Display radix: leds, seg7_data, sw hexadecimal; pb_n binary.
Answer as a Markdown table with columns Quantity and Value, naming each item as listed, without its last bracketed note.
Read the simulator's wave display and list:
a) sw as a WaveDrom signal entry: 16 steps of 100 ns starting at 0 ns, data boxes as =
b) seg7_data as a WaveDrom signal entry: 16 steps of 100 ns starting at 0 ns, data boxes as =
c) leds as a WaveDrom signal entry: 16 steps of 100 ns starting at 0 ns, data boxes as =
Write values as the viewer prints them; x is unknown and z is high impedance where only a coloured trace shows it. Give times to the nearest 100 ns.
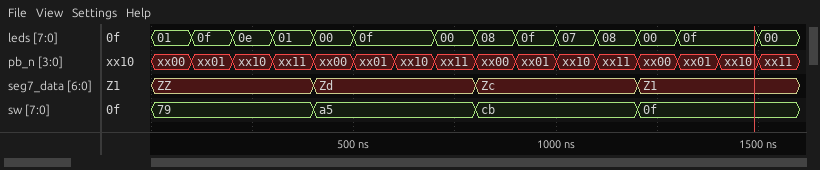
| Quantity | Value |
|---|---|
| sw as a WaveDrom signal entry: 16 steps of 100 ns starting at 0 ns, data boxes as = | {name: 'sw', wave: '=...=...=...=...', data: '79 a5 cb 0f'} |
| seg7_data as a WaveDrom signal entry: 16 steps of 100 ns starting at 0 ns, data boxes as = | {name: 'seg7_data', wave: '=...=...=...=...', data: 'ZZ Zd Zc Z1'} |
| leds as a WaveDrom signal entry: 16 steps of 100 ns starting at 0 ns, data boxes as = | {name: 'leds', wave: '======.=======.=', data: '01 0f 0e 01 00 0f 00 08 0f 07 08 00 0f 00'} |
